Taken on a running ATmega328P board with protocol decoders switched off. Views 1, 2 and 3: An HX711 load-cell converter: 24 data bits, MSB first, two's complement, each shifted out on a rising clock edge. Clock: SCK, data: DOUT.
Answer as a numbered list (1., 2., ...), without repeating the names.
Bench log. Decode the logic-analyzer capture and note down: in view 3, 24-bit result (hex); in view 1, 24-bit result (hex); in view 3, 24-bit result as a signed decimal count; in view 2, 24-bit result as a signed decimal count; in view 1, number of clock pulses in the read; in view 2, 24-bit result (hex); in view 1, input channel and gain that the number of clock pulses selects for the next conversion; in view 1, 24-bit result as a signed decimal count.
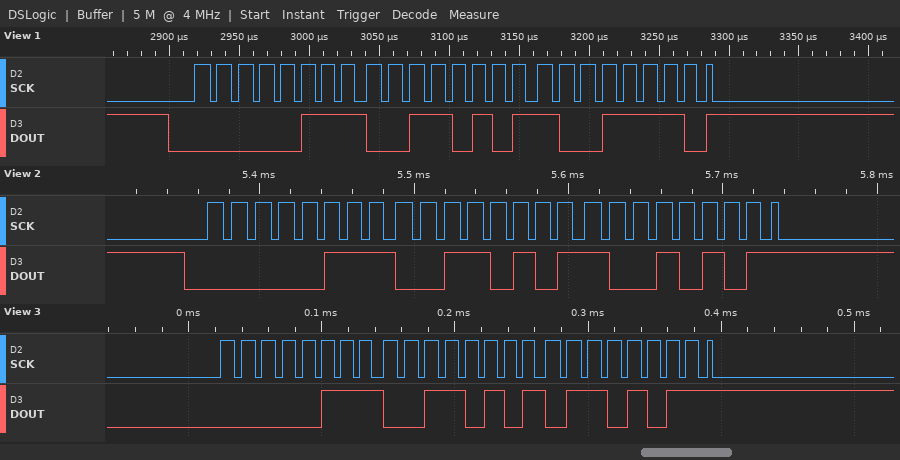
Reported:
1. 0x07356B
2. 0x07359E
3. 472427
4. 472469
5. 25
6. 0x073595
7. channel A, gain 128
8. 472478
